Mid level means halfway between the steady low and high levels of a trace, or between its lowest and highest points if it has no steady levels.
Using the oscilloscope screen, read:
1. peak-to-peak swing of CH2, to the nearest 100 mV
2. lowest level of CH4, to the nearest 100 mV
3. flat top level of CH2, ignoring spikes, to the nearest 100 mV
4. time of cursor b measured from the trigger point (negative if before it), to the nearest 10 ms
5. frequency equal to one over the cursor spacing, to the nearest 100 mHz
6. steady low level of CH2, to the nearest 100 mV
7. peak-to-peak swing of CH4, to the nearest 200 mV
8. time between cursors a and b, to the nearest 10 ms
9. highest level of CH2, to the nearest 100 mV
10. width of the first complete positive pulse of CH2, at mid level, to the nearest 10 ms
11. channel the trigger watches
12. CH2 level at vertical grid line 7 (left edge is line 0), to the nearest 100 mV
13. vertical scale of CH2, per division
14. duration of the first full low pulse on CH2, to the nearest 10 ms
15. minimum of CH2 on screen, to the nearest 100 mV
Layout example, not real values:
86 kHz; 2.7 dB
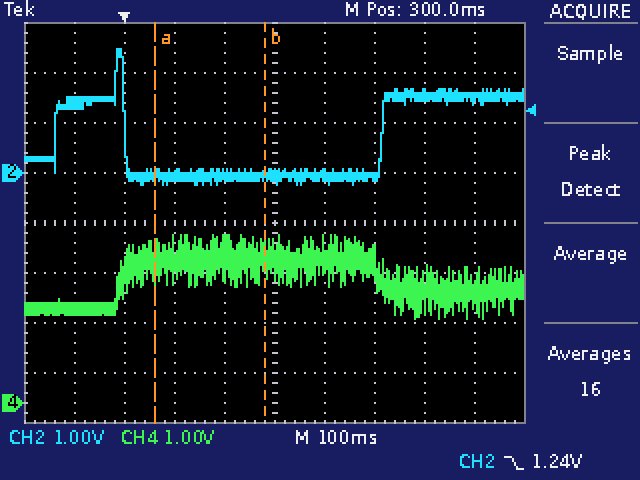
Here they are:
2.7 V; 1.7 V; 1.5 V; +280 ms; 4.5 Hz; -100 mV; 1.6 V; 220 ms; 2.5 V; 140 ms; CH2; -100 mV; 1 V; 510 ms; -200 mV
